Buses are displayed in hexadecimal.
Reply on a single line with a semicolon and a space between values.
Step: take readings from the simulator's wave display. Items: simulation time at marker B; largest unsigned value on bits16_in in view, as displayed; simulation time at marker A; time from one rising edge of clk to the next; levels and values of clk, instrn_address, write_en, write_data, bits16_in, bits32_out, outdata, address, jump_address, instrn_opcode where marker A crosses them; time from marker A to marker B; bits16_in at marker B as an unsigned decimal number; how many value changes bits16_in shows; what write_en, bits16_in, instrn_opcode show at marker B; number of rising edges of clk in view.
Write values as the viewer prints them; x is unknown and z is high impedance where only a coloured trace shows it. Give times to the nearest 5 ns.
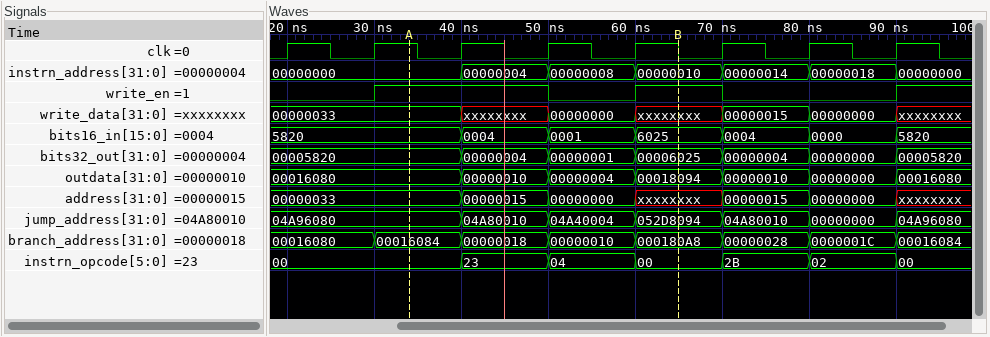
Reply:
65 ns; 6025; 35 ns; 10 ns; clk=1, instrn_address=00000000, write_en=1, write_data=00000033, bits16_in=5820, bits32_out=00005820, outdata=00016080, address=00000033, jump_address=04A96080, instrn_opcode=00; 30 ns; 24613; 6; write_en=1, bits16_in=6025, instrn_opcode=00; 8
